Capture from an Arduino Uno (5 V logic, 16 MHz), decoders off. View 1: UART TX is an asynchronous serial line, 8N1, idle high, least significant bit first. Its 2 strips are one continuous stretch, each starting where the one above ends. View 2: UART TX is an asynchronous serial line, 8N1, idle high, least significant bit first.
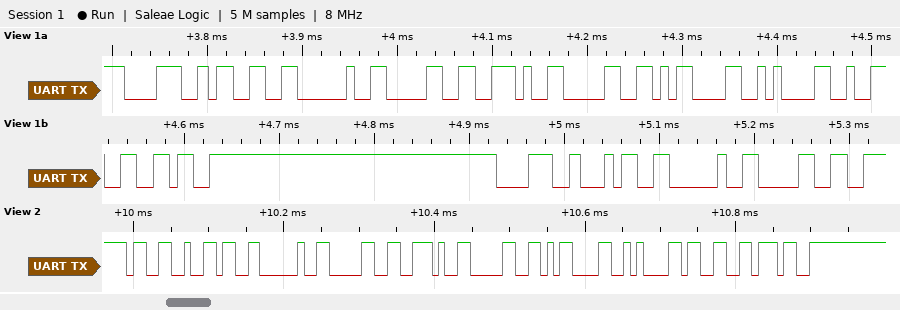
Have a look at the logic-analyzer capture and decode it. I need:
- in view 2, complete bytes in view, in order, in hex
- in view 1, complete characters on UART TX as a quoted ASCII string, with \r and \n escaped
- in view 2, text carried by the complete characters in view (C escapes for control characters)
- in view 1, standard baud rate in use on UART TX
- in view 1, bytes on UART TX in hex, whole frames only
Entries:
33 36 20 30 2E 30 0D 0A 33 37
"83 0.0\r\n2684 0"
"36 0.0\r\n37"
115200 baud
38 33 20 30 2E 30 0D 0A 32 36 38 34 20 30
